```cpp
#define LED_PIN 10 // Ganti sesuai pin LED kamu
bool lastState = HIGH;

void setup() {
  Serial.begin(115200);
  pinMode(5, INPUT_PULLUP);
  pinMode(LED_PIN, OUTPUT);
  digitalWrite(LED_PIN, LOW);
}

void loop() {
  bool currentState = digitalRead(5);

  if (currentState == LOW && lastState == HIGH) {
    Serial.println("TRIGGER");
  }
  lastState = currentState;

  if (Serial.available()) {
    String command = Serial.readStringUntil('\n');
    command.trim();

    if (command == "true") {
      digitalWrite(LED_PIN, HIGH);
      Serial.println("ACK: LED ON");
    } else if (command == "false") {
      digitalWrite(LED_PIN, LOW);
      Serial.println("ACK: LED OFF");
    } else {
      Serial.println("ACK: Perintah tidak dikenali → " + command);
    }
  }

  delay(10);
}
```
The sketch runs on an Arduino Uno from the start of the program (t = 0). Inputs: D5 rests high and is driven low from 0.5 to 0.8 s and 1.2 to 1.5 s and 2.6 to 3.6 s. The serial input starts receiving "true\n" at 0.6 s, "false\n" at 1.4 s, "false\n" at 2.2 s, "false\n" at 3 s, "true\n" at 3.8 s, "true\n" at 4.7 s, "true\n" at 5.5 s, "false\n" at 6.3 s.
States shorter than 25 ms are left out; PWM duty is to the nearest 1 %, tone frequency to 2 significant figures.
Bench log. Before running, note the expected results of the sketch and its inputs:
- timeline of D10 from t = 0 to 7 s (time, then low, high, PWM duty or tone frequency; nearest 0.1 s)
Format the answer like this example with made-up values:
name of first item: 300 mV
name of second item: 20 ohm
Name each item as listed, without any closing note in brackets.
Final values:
timeline of D10 from t = 0 to 7 s: 0 s low; 0.6 s high; 1.4 s low; 3.8 s high; 6.3 s low
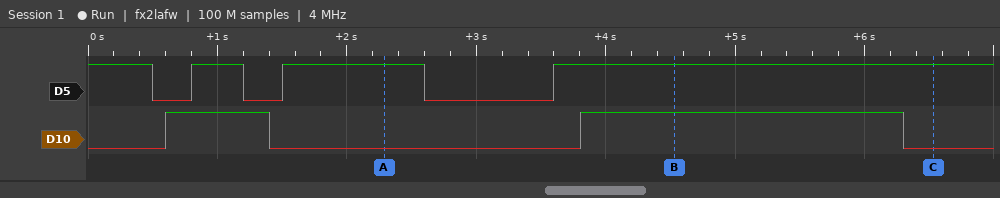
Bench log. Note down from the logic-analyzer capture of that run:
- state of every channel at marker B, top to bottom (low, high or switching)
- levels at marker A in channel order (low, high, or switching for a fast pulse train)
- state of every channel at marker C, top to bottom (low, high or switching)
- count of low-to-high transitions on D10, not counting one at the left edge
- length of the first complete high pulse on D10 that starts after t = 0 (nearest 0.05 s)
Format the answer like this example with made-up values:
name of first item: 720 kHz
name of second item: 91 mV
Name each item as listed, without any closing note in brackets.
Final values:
state of every channel at marker B, top to bottom: D5 high, D10 high
levels at marker A in channel order: D5 high, D10 low
state of every channel at marker C, top to bottom: D5 high, D10 low
count of low-to-high transitions on D10, not counting one at the left edge: 2
length of the first complete high pulse on D10 that starts after t = 0: 0.80 s
